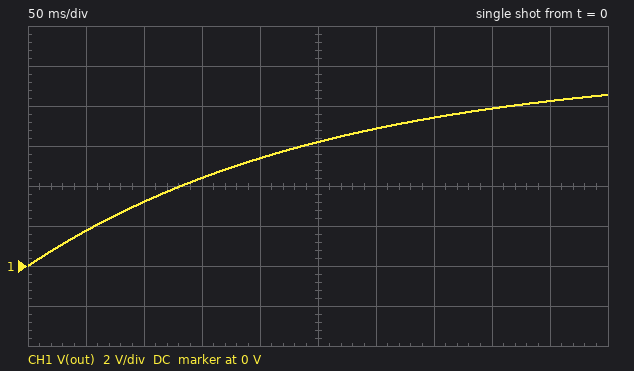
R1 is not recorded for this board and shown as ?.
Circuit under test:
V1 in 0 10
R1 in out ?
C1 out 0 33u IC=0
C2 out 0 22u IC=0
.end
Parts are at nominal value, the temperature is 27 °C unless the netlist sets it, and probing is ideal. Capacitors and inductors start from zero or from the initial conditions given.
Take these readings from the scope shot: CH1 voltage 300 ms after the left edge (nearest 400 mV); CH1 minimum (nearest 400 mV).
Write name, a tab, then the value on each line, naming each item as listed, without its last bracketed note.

CH1 voltage 300 ms after the left edge	6.8 V
CH1 minimum	0 V
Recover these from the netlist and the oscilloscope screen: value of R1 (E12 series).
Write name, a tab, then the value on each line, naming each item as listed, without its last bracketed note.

value of R1	4.7 kΩ
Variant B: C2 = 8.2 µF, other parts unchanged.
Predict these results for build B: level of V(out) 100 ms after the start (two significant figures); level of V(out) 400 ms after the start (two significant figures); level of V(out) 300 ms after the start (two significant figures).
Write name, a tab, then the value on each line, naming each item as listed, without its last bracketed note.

level of V(out) 100 ms after the start	4.0 V
level of V(out) 400 ms after the start	8.7 V
level of V(out) 300 ms after the start	7.9 V
